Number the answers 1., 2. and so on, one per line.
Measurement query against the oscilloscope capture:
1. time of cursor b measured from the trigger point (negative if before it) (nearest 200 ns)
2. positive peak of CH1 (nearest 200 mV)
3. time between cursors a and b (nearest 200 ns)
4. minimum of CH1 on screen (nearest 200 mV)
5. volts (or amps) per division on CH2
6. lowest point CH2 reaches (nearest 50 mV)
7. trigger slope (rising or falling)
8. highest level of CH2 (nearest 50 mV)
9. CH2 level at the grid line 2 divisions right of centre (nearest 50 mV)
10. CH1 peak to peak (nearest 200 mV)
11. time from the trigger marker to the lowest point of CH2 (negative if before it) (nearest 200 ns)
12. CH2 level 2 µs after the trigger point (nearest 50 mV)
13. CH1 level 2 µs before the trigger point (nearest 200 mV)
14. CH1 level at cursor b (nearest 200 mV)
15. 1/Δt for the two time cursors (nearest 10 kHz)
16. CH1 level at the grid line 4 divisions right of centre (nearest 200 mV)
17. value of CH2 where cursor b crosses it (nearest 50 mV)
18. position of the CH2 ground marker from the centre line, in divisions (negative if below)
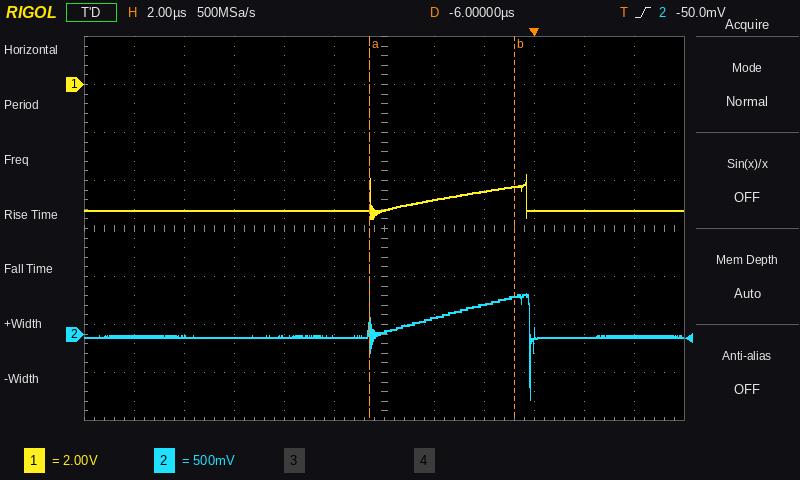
1. -800 ns
2. -3.8 V
3. 5.8 µs
4. -5.6 V
5. 500 mV
6. -700 mV
7. rising
8. 500 mV
9. 300 mV
10. 1.8 V
11. -200 ns
12. -50 mV
13. -4.4 V
14. -4.2 V
15. 170 kHz
16. -5.2 V
17. 400 mV
18. -2.2 div
